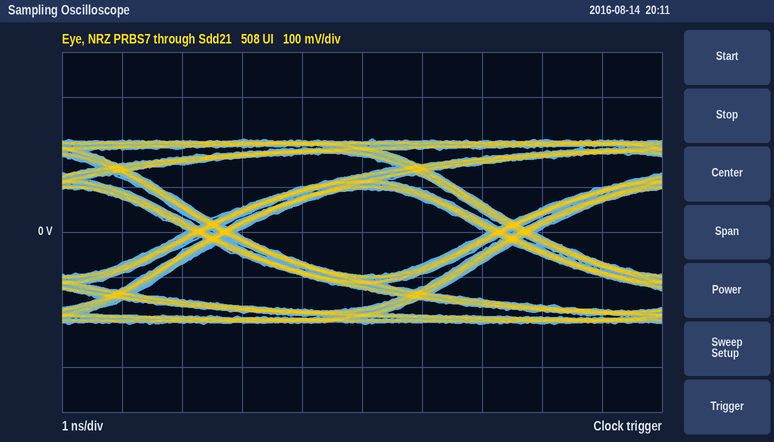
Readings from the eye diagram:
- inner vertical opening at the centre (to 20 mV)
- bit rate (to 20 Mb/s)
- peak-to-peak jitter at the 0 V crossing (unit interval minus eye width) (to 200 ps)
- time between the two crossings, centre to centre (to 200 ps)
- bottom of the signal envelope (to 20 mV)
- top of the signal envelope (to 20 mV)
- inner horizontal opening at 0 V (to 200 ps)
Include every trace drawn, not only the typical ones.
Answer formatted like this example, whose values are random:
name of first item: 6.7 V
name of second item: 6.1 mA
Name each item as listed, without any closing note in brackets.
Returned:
inner vertical opening at the centre: 200 mV
bit rate: 200 Mb/s
peak-to-peak jitter at the 0 V crossing (unit interval minus eye width): 800 ps
time between the two crossings, centre to centre: 5.0 ns
bottom of the signal envelope: -200 mV
top of the signal envelope: 200 mV
inner horizontal opening at 0 V: 4.2 ns
